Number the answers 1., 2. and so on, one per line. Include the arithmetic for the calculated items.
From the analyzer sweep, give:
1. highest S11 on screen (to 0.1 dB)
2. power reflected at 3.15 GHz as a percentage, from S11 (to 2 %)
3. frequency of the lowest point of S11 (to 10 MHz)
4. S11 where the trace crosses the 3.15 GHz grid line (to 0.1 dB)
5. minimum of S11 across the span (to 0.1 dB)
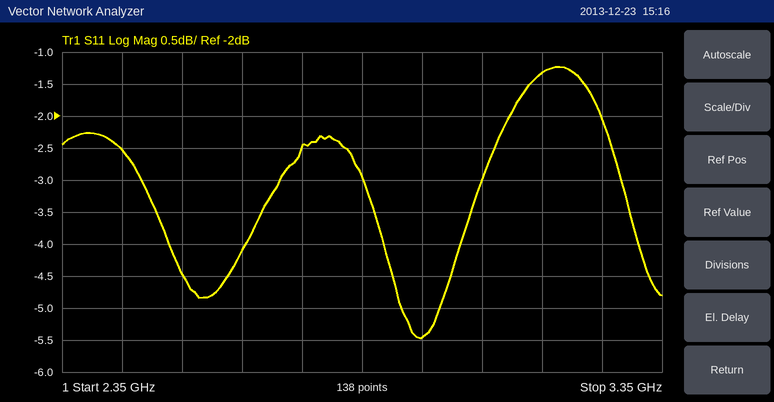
1. -1.2 dB
2. 10^(-1.3/10) ≈ 74 %
3. 2.95 GHz
4. -1.3 dB
5. -5.5 dB
